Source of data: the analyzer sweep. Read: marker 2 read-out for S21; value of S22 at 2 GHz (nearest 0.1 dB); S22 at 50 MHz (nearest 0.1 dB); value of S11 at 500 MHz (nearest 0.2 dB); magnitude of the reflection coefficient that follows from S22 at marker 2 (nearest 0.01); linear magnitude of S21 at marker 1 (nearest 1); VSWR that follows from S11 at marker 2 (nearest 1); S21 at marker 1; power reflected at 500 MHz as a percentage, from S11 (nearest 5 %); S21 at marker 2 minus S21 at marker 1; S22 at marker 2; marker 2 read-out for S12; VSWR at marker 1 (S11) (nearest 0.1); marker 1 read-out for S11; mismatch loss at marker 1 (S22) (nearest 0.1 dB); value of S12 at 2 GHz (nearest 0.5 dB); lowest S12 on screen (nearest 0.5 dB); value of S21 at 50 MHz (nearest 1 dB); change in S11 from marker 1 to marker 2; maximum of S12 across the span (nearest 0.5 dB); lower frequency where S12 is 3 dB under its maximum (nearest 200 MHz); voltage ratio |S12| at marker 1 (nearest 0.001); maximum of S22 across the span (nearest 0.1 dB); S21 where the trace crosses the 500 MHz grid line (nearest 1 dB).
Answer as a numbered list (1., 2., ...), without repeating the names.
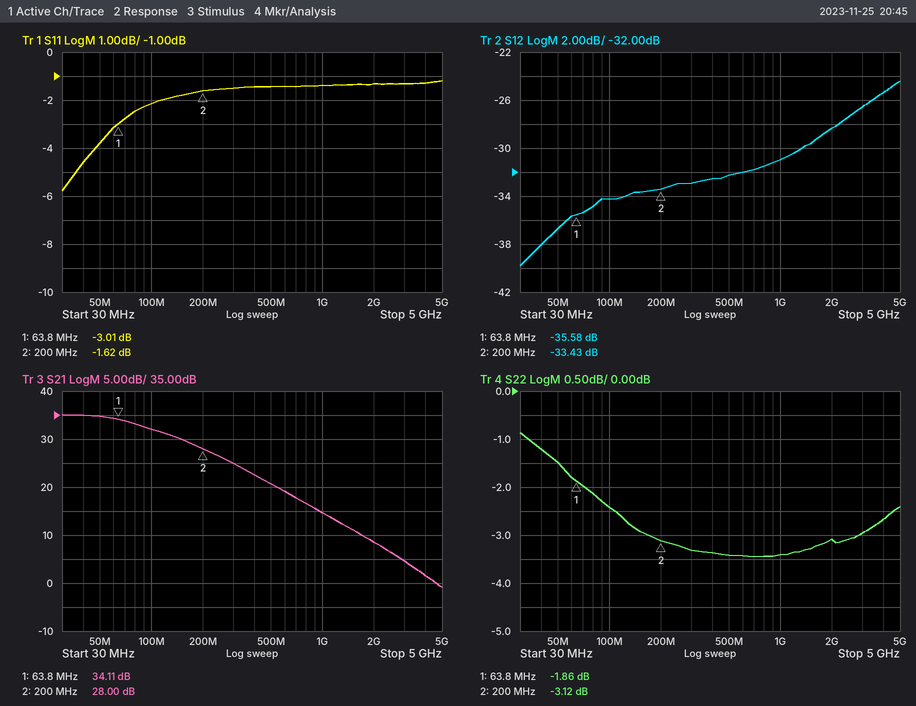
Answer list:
1. 28.00 dB
2. -3.1 dB
3. -1.5 dB
4. -1.4 dB
5. 0.70
6. 51
7. 11
8. 34.11 dB
9. 70 %
10. -6.11 dB
11. -3.12 dB
12. -33.43 dB
13. 5.8
14. -3.01 dB
15. 4.6 dB
16. -28.5 dB
17. -40.0 dB
18. 35 dB
19. 1.39 dB
20. -24.5 dB
21. 2.4 GHz
22. 0.017
23. -0.9 dB
24. 21 dB
